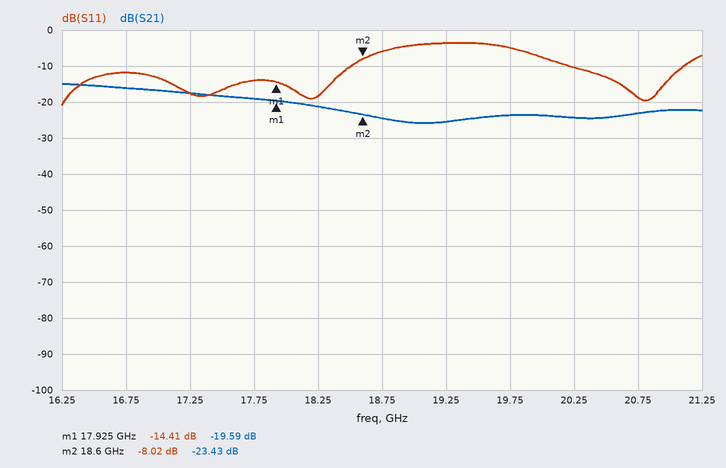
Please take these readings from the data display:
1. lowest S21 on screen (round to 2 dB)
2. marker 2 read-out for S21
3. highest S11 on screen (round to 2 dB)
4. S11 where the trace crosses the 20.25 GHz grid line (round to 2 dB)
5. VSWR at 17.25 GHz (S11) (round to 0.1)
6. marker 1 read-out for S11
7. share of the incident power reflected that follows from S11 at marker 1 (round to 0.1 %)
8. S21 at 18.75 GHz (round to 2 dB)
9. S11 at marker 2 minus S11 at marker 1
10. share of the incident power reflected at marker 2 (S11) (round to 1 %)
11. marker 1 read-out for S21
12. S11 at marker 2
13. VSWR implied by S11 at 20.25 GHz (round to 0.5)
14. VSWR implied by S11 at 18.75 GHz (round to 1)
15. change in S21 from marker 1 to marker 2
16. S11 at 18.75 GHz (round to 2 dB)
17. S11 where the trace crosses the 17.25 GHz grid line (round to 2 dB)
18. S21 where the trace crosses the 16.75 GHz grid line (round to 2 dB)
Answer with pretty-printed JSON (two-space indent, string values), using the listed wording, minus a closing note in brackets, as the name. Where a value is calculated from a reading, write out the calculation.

{
  "lowest S21 on screen": "-26 dB",
  "marker 2 read-out for S21": "-23.43 dB",
  "highest S11 on screen": "-4 dB",
  "S11 where the trace crosses the 20.25 GHz grid line": "-10 dB",
  "VSWR at 17.25 GHz (S11)": "|Γ| = 10^(-18/20) = 0.1259; VSWR = (1 + 0.1259)/(1 − 0.1259) ≈ 1.3",
  "marker 1 read-out for S11": "-14.41 dB",
  "share of the incident power reflected that follows from S11 at marker 1": "10^(-14.41/10) ≈ 3.6 %",
  "S21 at 18.75 GHz": "-24 dB",
  "S11 at marker 2 minus S11 at marker 1": "-8.02 − (-14.41) = 6.39 dB",
  "share of the incident power reflected at marker 2 (S11)": "10^(-8.02/10) ≈ 16 %",
  "marker 1 read-out for S21": "-19.59 dB",
  "S11 at marker 2": "-8.02 dB",
  "VSWR implied by S11 at 20.25 GHz": "|Γ| = 10^(-10/20) = 0.3162; VSWR = (1 + 0.3162)/(1 − 0.3162) ≈ 1.92, so 2.0 to the nearest 0.5",
  "VSWR implied by S11 at 18.75 GHz": "|Γ| = 10^(-6/20) = 0.5012; VSWR = (1 + 0.5012)/(1 − 0.5012) ≈ 3",
  "change in S21 from marker 1 to marker 2": "-23.43 − (-19.59) = -3.84 dB",
  "S11 at 18.75 GHz": "-6 dB",
  "S11 where the trace crosses the 17.25 GHz grid line": "-18 dB",
  "S21 where the trace crosses the 16.75 GHz grid line": "-16 dB"
}
